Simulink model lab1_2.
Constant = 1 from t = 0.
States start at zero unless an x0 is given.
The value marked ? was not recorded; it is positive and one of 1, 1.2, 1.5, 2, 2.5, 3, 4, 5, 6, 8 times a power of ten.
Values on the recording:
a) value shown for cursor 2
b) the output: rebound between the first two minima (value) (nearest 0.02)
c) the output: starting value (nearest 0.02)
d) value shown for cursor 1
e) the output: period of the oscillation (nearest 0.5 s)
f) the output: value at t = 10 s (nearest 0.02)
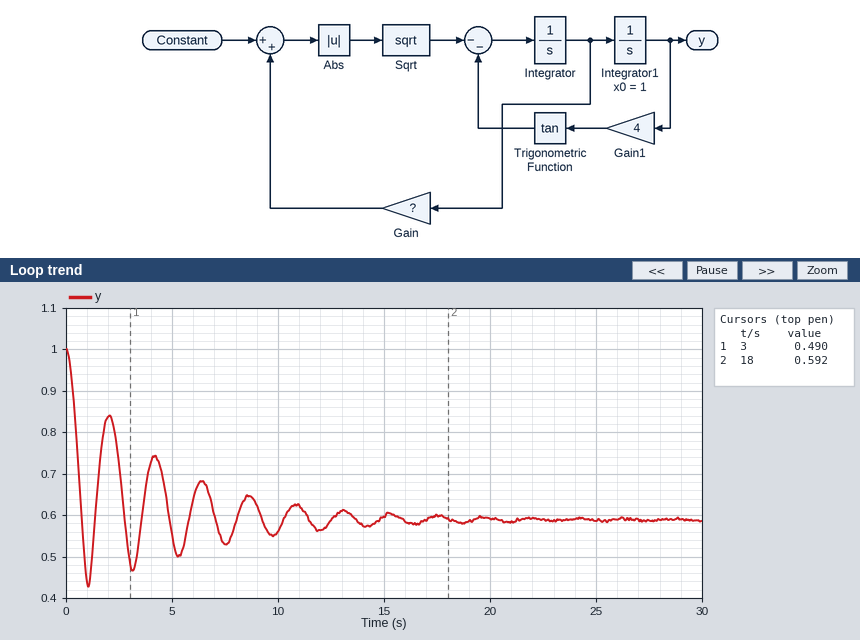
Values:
0.592
0.84
1.00
0.490
2.0 s
0.56
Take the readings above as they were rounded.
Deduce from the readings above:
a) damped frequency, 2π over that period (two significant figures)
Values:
3.1 rad/s
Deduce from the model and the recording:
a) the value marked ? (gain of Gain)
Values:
0.8
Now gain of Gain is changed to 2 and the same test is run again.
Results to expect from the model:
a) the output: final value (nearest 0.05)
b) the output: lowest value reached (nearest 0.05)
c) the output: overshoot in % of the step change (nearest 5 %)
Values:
0.60
0.45
35 %
